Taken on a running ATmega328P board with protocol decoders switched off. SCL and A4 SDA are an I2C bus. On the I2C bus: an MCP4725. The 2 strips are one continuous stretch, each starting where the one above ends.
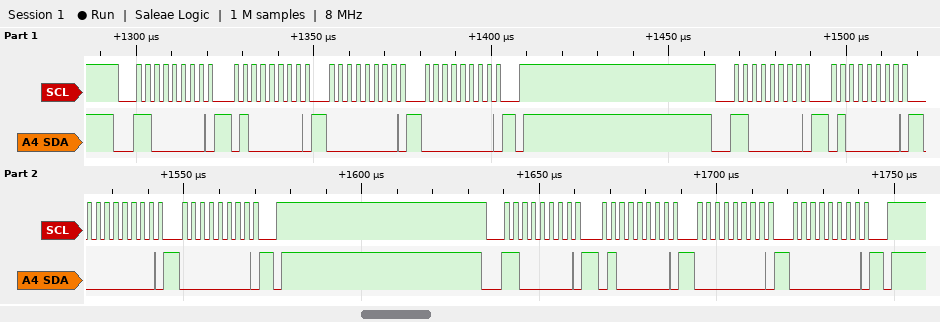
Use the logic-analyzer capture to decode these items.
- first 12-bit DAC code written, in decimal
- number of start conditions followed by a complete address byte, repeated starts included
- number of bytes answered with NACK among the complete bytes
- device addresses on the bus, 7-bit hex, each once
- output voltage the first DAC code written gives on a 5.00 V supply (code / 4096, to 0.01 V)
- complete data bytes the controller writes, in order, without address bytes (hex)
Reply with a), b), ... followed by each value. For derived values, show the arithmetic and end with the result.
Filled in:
a) 0
b) 3
c) 0
d) 0x60
e) 0 / 4096 x 5.00 V = 0.00 V
f) 40 00 00 40 00 00 40 00 00
